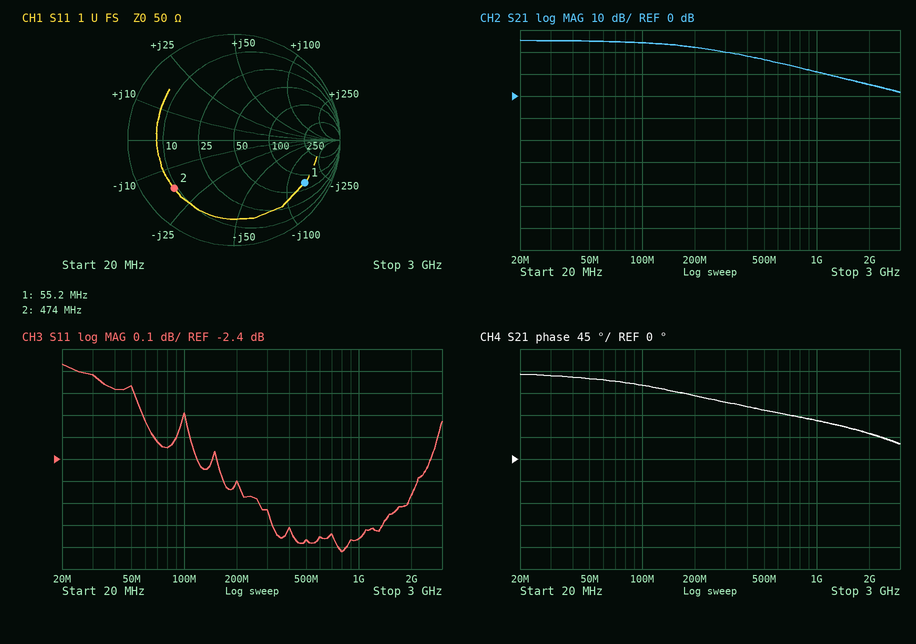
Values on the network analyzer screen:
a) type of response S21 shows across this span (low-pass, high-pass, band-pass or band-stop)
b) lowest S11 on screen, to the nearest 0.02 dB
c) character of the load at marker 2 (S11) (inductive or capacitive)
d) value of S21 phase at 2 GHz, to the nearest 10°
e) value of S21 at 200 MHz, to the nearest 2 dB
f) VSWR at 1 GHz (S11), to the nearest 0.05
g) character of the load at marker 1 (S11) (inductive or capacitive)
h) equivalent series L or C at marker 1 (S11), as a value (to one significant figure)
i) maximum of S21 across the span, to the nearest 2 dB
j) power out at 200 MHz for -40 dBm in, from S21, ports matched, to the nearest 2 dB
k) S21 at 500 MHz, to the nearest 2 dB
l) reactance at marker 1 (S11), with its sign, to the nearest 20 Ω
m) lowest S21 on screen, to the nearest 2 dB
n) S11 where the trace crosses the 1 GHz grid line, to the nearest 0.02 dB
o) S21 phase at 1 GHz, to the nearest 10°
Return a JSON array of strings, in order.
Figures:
["low-pass", "-2.82 dB", "capacitive", "50°", "22 dB", "6.35", "capacitive", "20 pF", "26 dB", "-18 dBm", "16 dB", "-140 Ω", "2 dB", "-2.76 dB", "80°"]
